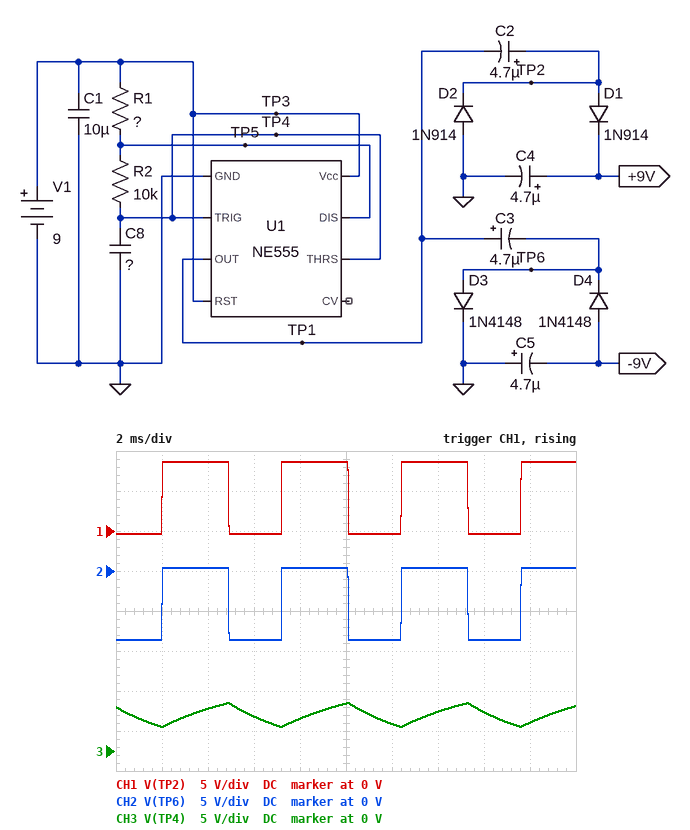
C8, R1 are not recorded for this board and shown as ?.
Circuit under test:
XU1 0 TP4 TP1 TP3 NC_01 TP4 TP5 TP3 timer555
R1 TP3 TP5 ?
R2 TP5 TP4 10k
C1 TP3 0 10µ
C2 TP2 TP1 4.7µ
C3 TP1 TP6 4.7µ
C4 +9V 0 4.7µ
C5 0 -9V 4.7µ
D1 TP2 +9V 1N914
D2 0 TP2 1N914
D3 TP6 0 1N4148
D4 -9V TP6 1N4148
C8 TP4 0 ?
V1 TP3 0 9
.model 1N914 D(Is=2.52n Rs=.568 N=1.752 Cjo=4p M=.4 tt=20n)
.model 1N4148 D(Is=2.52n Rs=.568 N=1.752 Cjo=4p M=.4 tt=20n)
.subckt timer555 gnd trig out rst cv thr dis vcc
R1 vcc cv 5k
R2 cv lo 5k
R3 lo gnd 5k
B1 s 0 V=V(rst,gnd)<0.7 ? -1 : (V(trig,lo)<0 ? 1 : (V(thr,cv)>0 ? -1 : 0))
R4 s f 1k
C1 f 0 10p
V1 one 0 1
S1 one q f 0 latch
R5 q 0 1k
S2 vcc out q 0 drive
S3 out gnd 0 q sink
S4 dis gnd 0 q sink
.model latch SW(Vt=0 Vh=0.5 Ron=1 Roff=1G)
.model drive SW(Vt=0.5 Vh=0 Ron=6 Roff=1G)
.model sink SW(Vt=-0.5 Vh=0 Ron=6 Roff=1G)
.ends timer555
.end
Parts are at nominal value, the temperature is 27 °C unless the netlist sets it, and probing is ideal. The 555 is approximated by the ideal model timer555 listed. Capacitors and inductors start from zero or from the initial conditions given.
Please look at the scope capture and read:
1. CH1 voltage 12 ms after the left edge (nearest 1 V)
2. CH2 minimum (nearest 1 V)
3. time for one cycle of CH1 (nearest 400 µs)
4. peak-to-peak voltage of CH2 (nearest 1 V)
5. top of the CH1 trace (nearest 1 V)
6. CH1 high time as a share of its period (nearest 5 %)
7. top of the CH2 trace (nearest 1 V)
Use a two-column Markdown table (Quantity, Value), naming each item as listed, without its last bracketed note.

| Quantity | Value |
|---|---|
| CH1 voltage 12 ms after the left edge | 0 V |
| CH2 minimum | -9 V |
| time for one cycle of CH1 | 5.2 ms |
| peak-to-peak voltage of CH2 | 9 V |
| top of the CH1 trace | 9 V |
| CH1 high time as a share of its period | 55 % |
| top of the CH2 trace | 0 V |
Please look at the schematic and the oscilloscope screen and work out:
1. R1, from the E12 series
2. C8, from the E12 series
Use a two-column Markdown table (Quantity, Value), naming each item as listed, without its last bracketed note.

| Quantity | Value |
|---|---|
| R1, from the E12 series | 2.7 kΩ |
| C8, from the E12 series | 330 nF |
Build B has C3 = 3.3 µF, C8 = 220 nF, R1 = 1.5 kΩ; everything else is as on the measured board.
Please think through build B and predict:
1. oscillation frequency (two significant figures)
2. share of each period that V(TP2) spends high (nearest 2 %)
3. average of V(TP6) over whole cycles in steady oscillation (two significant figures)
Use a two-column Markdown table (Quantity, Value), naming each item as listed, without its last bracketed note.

| Quantity | Value |
|---|---|
| oscillation frequency | 300 Hz |
| share of each period that V(TP2) spends high | 54 % |
| average of V(TP6) over whole cycles in steady oscillation | -3.9 V |
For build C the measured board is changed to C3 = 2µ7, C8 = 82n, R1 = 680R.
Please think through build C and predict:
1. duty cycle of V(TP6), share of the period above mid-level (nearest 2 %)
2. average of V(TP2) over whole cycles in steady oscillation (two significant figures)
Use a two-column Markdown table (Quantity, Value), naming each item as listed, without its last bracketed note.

| Quantity | Value |
|---|---|
| duty cycle of V(TP6), share of the period above mid-level | 52 % |
| average of V(TP2) over whole cycles in steady oscillation | 4.3 V |
